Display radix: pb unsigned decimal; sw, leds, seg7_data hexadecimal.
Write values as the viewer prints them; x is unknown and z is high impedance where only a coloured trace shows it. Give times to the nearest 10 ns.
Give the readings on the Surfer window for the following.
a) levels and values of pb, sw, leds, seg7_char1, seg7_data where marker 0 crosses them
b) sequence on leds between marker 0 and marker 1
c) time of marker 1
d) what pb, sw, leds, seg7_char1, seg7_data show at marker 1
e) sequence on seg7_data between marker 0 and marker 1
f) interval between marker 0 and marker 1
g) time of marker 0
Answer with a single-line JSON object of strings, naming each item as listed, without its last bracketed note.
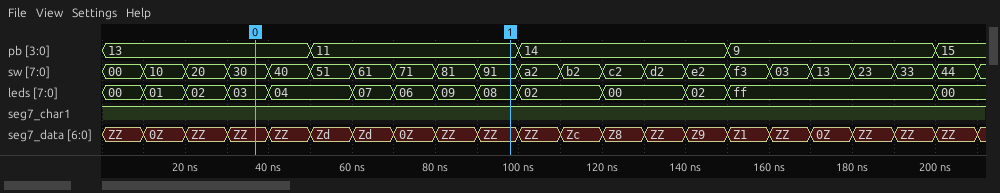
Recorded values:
{"levels and values of pb, sw, leds, seg7_char1, seg7_data where marker 0 crosses them": "pb=13, sw=30, leds=03, seg7_char1=1, seg7_data=ZZ", "sequence on leds between marker 0 and marker 1": "03, 04, 07, 06, 09, 08", "time of marker 1": "100 ns", "what pb, sw, leds, seg7_char1, seg7_data show at marker 1": "pb=11, sw=91, leds=08, seg7_char1=1, seg7_data=ZZ", "sequence on seg7_data between marker 0 and marker 1": "ZZ, ZZ, Zd, Zd, 0Z, ZZ, ZZ", "interval between marker 0 and marker 1": "60 ns", "time of marker 0": "40 ns"}
